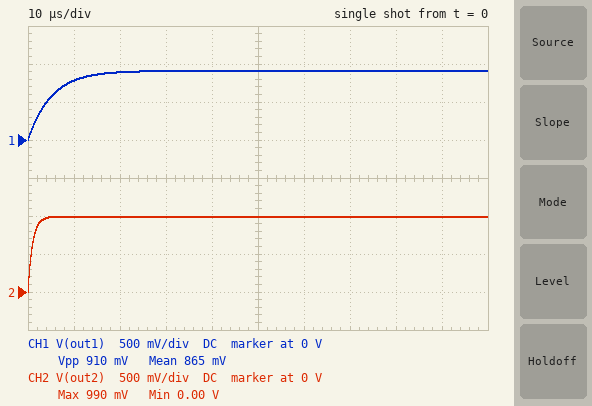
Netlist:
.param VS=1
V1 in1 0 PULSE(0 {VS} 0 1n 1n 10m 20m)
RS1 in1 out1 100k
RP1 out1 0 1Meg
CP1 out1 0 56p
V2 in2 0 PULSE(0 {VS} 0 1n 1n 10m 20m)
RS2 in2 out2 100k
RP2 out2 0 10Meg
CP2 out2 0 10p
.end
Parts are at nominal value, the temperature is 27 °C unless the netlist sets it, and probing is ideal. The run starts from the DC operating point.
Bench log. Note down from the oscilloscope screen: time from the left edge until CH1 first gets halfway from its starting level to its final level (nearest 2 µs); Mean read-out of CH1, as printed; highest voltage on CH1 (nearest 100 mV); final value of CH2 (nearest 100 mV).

4 µs
865 mV
900 mV
1.0 V
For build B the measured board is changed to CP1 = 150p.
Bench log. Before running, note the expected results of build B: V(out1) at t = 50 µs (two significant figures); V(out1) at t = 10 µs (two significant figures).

890 mV
470 mV
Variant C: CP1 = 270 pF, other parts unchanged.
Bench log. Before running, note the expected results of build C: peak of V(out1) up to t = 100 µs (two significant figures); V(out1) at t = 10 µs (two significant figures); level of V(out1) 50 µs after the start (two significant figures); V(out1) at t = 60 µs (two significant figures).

890 mV
300 mV
790 mV
830 mV
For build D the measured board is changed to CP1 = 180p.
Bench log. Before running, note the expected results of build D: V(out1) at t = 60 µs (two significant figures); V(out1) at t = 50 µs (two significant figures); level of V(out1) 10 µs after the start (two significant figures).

890 mV
870 mV
420 mV
